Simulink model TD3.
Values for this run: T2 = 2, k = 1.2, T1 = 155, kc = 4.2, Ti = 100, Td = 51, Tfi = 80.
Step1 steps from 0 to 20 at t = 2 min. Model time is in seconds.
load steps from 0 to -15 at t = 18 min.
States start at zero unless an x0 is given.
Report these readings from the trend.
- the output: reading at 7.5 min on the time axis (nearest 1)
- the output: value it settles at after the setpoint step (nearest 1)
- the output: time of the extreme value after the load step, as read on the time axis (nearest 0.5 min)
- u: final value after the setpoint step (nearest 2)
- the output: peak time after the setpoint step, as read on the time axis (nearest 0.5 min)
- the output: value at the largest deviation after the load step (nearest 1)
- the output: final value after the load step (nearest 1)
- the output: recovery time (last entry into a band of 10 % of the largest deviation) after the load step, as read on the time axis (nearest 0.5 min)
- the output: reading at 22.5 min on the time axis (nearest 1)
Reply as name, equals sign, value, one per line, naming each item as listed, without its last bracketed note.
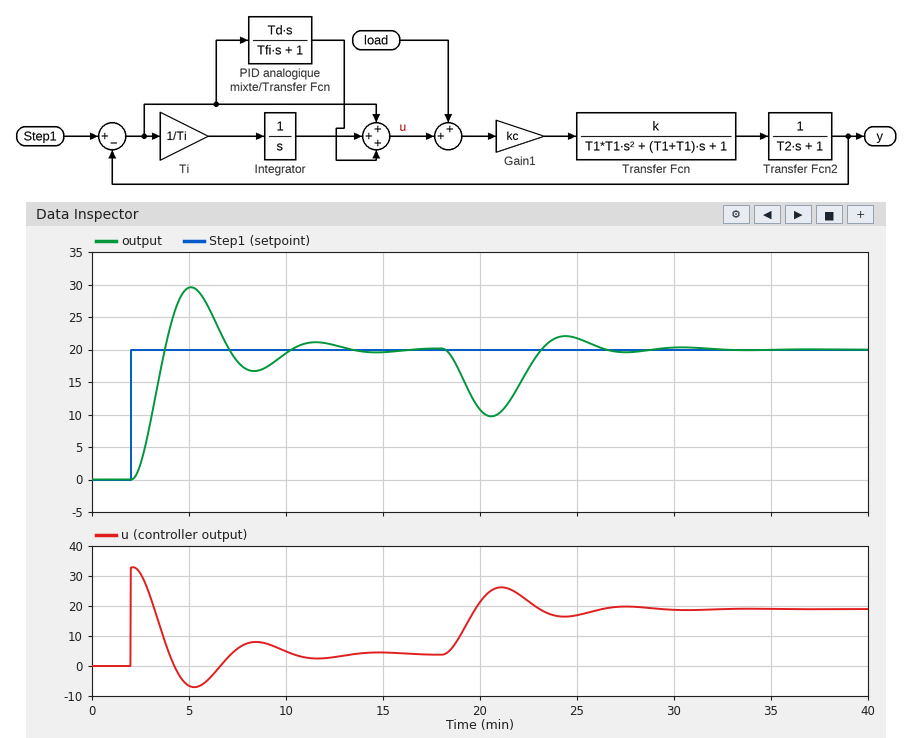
the output: reading at 7.5 min on the time axis = 18
the output: value it settles at after the setpoint step = 20
the output: time of the extreme value after the load step, as read on the time axis = 20.5 min
u: final value after the setpoint step = 4
the output: peak time after the setpoint step, as read on the time axis = 5.0 min
the output: value at the largest deviation after the load step = 10
the output: final value after the load step = 20
the output: recovery time (last entry into a band of 10 % of the largest deviation) after the load step, as read on the time axis = 25.5 min
the output: reading at 22.5 min on the time axis = 17
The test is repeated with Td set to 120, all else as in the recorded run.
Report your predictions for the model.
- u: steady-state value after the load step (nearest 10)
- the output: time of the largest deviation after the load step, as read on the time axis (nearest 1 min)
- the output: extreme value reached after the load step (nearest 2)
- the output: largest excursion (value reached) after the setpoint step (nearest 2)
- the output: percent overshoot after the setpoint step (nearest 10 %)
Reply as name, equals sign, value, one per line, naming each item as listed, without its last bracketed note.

u: steady-state value after the load step = 20
the output: time of the largest deviation after the load step, as read on the time axis = 20 min
the output: extreme value reached after the load step = 12
the output: largest excursion (value reached) after the setpoint step = 26
the output: percent overshoot after the setpoint step = 30 %
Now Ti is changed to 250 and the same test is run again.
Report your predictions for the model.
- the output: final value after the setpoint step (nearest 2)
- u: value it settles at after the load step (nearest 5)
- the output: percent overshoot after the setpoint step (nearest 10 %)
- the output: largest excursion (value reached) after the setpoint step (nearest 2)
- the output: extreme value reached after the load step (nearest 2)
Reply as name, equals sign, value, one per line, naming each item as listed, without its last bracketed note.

the output: final value after the setpoint step = 20
u: value it settles at after the load step = 20
the output: percent overshoot after the setpoint step = 20 %
the output: largest excursion (value reached) after the setpoint step = 24
the output: extreme value reached after the load step = 8
